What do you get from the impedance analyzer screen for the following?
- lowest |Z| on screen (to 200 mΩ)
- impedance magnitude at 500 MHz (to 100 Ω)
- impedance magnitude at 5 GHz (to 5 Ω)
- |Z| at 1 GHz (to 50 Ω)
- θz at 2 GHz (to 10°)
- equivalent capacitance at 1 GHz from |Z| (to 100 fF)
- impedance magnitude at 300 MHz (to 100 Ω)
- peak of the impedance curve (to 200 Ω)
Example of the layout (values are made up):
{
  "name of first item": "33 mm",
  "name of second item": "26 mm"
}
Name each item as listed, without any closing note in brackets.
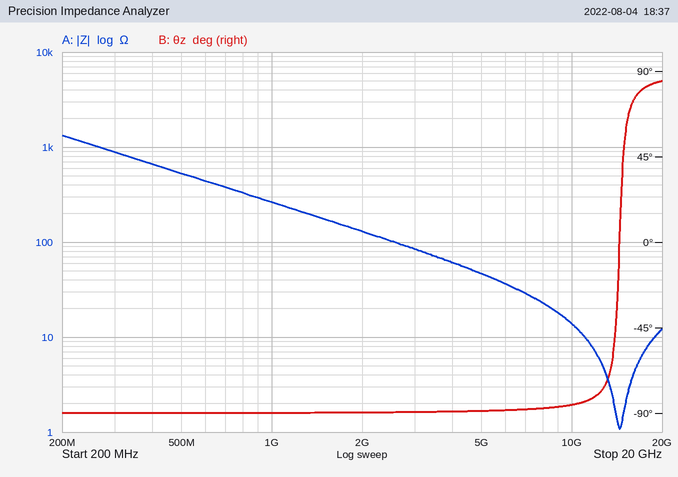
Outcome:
{
  "lowest |Z| on screen": "1.0 Ω",
  "impedance magnitude at 500 MHz": "500 Ω",
  "impedance magnitude at 5 GHz": "45 Ω",
  "|Z| at 1 GHz": "250 Ω",
  "θz at 2 GHz": "-90°",
  "equivalent capacitance at 1 GHz from |Z|": "600 fF",
  "impedance magnitude at 300 MHz": "900 Ω",
  "peak of the impedance curve": "1.4 kΩ"
}
